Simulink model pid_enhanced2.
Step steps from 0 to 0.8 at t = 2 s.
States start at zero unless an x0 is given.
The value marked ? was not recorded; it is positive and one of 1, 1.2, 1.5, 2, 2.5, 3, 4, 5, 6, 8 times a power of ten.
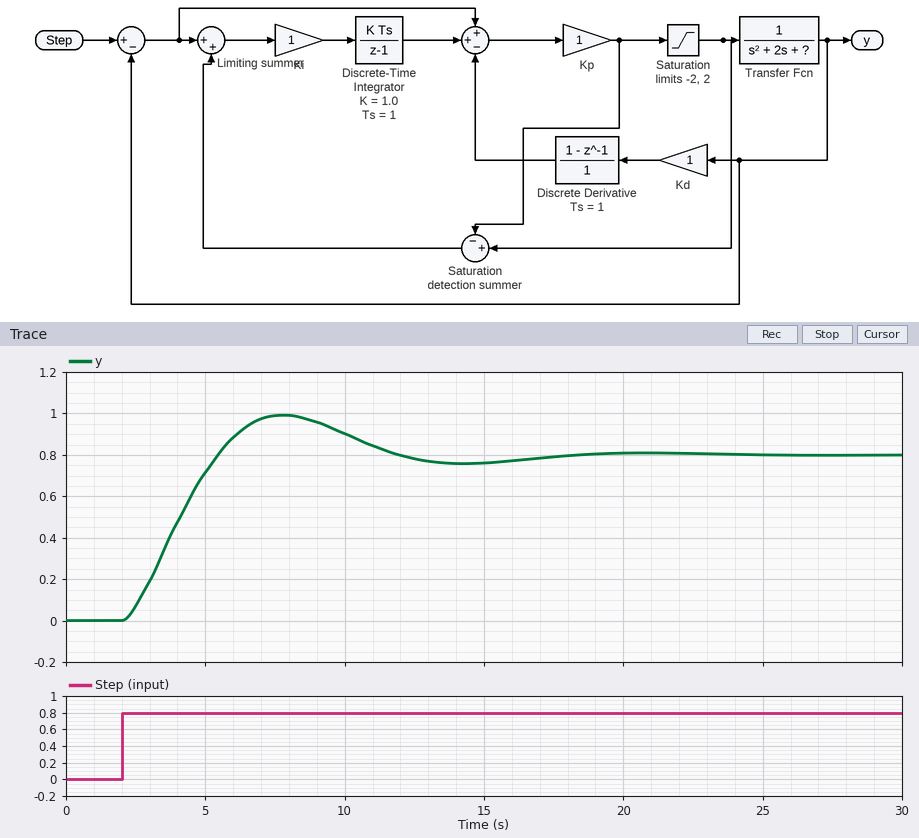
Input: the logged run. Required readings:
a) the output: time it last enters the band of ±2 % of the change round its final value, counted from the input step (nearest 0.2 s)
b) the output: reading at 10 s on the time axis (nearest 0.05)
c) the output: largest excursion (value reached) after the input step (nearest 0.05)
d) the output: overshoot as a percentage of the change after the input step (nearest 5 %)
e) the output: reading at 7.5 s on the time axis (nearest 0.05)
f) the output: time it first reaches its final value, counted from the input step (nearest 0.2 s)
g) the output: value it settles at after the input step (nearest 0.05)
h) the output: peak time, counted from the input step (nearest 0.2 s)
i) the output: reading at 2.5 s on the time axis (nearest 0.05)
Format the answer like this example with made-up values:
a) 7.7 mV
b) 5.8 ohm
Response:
a) 15.0 s
b) 0.90
c) 1.00
d) 25 %
e) 1.00
f) 3.4 s
g) 0.80
h) 5.8 s
i) 0.05
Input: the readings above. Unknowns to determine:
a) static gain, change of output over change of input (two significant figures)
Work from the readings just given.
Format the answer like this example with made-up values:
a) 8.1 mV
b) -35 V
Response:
a) 1.0
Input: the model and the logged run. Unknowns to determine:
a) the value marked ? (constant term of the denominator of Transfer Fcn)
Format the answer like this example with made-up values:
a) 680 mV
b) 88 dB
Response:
a) 1.5
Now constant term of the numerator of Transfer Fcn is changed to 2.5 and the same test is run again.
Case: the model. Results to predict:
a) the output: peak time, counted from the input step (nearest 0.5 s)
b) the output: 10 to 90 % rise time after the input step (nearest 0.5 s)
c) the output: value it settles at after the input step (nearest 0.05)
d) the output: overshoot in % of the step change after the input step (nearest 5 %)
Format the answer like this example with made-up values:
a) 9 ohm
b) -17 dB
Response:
a) 4.0 s
b) 1.5 s
c) 0.80
d) 40 %
